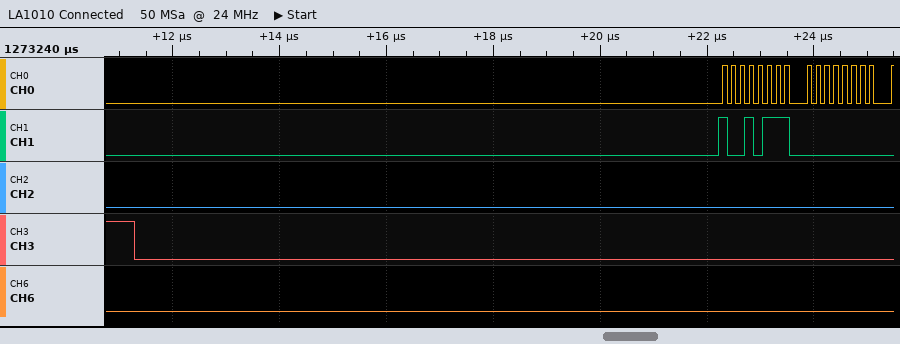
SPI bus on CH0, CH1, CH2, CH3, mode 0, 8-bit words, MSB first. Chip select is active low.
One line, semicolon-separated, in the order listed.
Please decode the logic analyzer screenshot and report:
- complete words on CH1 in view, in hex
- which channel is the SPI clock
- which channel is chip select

97, 00; CH0; CH3
